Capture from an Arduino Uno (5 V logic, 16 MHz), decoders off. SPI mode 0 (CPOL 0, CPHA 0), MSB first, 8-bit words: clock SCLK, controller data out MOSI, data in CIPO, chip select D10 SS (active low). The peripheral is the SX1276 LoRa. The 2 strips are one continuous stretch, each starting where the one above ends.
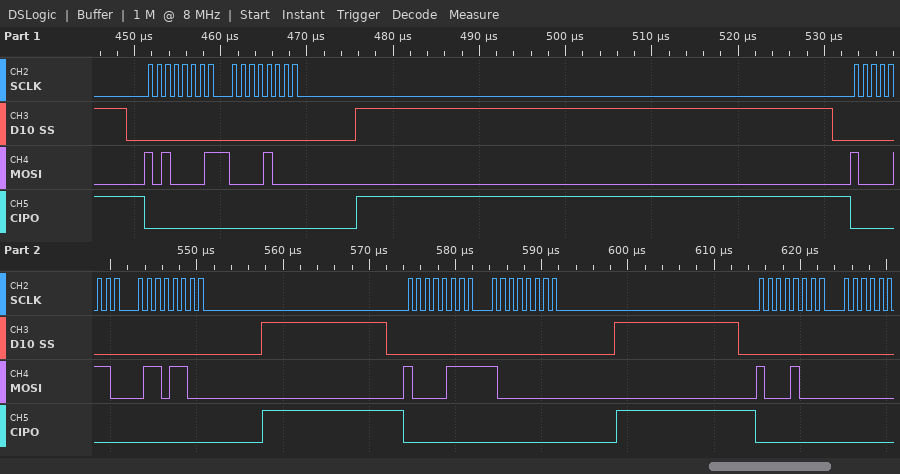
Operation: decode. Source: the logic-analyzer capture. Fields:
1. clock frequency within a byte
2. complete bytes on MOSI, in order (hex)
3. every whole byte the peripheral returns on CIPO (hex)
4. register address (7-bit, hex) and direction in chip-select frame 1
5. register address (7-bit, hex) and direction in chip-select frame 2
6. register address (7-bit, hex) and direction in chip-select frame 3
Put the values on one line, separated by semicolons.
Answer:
1 MHz; 0xA1 0x08 0x86 0x6C 0x87 0x80 0x88; 0x00 0x00 0x00 0x00 0x00 0x00 0x00; 0x21 write; 0x06 write; 0x07 write
